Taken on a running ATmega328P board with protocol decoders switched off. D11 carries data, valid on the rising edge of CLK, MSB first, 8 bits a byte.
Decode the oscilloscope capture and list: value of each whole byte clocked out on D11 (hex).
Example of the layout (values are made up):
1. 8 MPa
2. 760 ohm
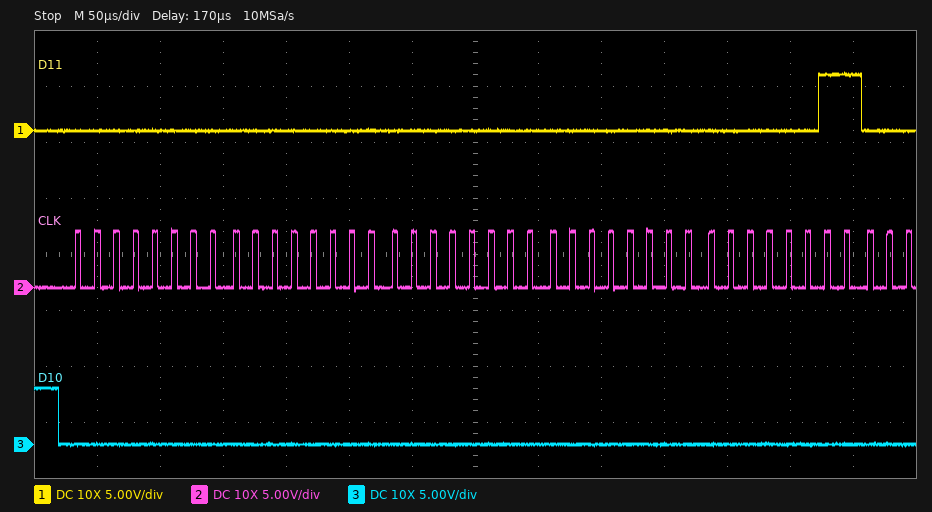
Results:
1. 00 00 00 00 03
